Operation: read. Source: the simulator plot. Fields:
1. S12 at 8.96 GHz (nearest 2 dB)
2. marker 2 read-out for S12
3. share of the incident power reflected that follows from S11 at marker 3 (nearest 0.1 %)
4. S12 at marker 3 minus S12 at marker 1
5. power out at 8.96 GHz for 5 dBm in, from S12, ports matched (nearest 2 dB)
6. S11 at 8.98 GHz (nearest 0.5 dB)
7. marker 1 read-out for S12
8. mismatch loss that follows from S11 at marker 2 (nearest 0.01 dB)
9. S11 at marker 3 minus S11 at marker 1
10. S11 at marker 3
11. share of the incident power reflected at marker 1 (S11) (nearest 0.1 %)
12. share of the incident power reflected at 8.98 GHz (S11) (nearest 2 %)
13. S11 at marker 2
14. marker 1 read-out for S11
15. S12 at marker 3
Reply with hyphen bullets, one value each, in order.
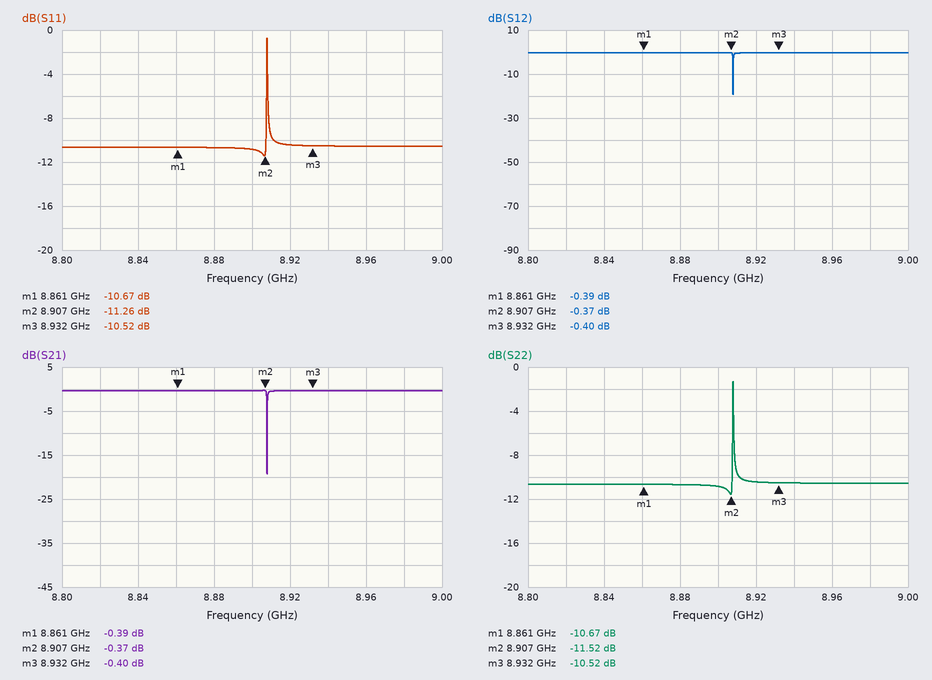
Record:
- 0 dB
- -0.37 dB
- 8.9 %
- -0.01 dB
- 4 dBm
- -10.5 dB
- -0.39 dB
- 0.34 dB
- 0.15 dB
- -10.52 dB
- 8.6 %
- 8 %
- -11.26 dB
- -10.67 dB
- -0.40 dB
